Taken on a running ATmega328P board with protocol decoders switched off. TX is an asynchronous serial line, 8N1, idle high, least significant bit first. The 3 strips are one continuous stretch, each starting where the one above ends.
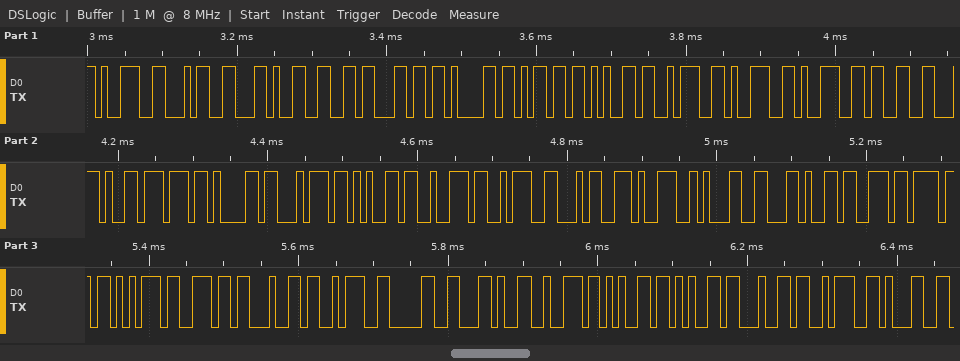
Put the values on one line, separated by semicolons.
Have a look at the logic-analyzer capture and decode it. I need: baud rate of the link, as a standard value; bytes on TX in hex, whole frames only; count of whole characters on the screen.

115200 baud; 39 34 2C 66 6C 61 6D 65 3A 39 39 33 2C 77 61 74 65 72 3A 34 39 31 2C 73 6F 75 6E 64 3A 30 2C 72 65 65 64 3A 31; 37
